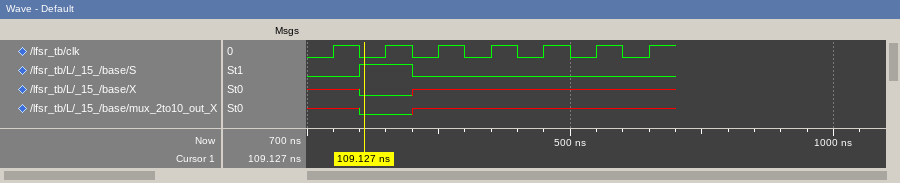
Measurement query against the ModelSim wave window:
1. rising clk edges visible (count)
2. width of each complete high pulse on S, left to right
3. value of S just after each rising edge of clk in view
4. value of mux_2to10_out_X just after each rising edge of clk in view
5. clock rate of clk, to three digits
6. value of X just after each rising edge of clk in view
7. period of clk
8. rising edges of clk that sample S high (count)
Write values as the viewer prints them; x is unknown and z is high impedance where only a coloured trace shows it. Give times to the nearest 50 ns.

7
100 ns
0 1 0 0 0 0 0
x 0 x x x x x
10.0 MHz
x 0 x x x x x
100 ns
1
